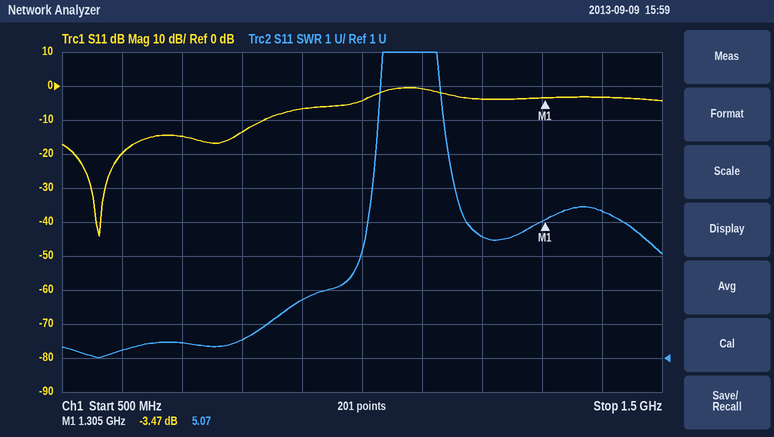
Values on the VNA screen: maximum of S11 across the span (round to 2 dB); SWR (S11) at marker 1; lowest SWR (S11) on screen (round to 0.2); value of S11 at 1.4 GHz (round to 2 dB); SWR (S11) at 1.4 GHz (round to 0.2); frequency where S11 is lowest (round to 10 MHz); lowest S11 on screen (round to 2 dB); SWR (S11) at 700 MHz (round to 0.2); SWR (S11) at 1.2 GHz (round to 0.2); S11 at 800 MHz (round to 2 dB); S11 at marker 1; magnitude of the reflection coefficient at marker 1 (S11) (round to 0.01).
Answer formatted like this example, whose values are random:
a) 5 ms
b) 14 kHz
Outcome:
a) 0 dB
b) 5.07
c) 1.0
d) -4 dB
e) 5.4
f) 560 MHz
g) -44 dB
h) 1.4
i) 4.6
j) -14 dB
k) -3.47 dB
l) 0.67
